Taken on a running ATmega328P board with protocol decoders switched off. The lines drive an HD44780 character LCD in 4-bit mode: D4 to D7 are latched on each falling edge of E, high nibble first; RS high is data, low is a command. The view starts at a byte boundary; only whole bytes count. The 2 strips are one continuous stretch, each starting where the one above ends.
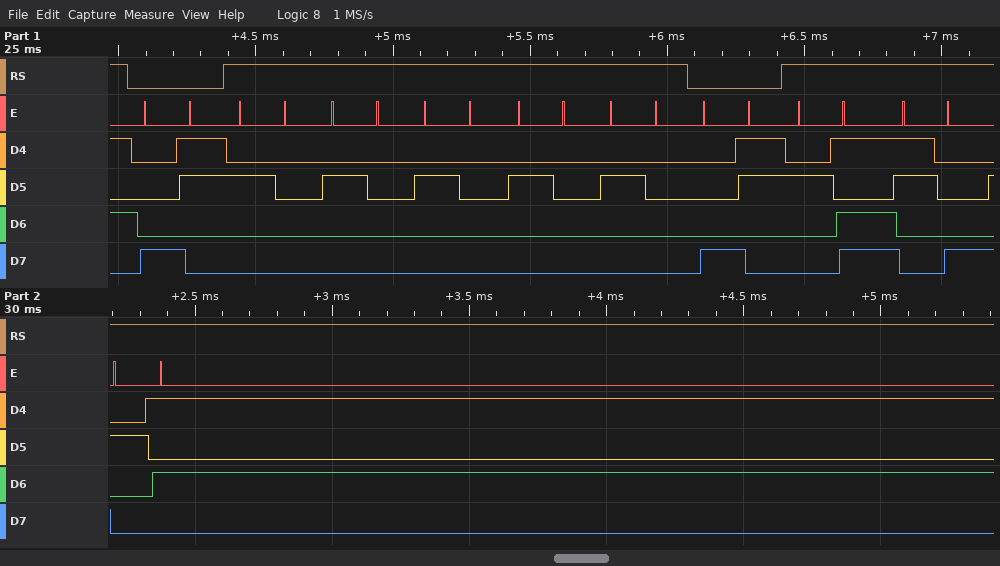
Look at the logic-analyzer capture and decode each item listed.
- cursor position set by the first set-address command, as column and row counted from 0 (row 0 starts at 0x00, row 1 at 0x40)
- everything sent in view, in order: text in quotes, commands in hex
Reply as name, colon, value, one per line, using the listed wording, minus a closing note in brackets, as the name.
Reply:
cursor position set by the first set-address command, as column and row counted from 0: column 3, row 0
everything sent in view, in order: text in quotes, commands in hex: 0x83 "     " 0x83 "-8%"
